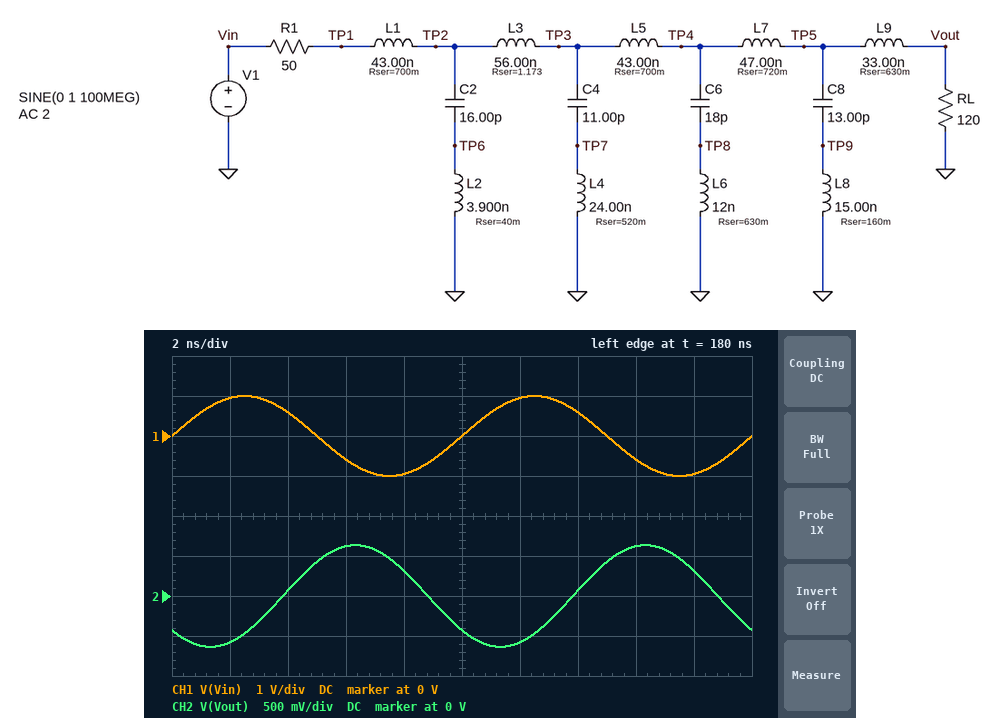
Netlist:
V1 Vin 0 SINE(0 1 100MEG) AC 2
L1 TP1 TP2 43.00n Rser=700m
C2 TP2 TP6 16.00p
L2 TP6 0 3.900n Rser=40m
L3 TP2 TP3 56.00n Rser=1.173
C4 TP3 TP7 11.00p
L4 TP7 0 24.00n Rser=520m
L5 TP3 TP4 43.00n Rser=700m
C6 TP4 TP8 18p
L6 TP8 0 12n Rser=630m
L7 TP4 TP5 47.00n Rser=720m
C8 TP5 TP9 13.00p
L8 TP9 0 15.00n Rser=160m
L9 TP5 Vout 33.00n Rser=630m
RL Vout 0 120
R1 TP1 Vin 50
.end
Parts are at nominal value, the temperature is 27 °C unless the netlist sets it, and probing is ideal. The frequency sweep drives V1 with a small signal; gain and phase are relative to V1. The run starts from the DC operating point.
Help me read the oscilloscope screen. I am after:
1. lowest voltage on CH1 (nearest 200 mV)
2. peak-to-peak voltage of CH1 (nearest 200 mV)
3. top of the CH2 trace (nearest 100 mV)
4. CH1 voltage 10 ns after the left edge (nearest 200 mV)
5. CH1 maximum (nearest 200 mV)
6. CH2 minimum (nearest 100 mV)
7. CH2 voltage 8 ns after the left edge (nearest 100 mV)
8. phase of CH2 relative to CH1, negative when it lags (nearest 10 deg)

-1.0 V
2.0 V
600 mV
0 V
1.0 V
-600 mV
300 mV
-140 deg
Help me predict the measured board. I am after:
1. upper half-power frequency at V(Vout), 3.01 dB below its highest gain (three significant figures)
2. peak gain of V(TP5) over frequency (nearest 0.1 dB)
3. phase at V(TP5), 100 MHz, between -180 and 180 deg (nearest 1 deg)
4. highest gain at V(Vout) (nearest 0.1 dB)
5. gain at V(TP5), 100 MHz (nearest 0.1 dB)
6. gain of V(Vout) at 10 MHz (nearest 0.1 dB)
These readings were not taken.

235 MHz
-2.8 dB
-128 deg
-2.9 dB
-3.8 dB
-3.2 dB
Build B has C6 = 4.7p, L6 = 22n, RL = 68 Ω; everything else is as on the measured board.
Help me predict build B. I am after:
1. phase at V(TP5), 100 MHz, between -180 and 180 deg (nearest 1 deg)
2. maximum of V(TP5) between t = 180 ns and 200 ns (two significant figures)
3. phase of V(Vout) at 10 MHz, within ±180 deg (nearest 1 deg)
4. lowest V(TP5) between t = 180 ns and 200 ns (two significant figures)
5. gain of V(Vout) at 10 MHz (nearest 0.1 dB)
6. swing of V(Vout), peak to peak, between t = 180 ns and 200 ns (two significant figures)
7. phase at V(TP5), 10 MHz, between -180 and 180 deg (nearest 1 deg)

-102 deg
590 mV
-11 deg
-590 mV
-5.1 dB
1.1 V
-10 deg
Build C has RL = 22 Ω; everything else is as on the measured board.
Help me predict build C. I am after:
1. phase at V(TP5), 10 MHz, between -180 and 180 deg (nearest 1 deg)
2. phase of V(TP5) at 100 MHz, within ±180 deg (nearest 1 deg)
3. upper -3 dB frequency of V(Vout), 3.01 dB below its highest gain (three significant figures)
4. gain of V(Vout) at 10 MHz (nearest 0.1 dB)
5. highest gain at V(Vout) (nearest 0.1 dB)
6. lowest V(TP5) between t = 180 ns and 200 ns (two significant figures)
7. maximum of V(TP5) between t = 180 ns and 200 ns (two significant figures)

-9 deg
-94 deg
249 MHz
-10.8 dB
-10.2 dB
-430 mV
430 mV
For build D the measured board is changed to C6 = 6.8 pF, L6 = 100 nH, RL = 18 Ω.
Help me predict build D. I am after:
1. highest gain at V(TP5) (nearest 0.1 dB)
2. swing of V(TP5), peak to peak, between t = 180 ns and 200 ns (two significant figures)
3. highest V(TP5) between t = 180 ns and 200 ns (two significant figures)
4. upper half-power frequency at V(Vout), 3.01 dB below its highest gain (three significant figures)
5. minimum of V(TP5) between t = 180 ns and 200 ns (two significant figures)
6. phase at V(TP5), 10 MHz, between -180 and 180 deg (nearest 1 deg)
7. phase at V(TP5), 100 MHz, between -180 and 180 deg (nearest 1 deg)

-5.9 dB
750 mV
380 mV
174 MHz
-380 mV
-7 deg
-74 deg
